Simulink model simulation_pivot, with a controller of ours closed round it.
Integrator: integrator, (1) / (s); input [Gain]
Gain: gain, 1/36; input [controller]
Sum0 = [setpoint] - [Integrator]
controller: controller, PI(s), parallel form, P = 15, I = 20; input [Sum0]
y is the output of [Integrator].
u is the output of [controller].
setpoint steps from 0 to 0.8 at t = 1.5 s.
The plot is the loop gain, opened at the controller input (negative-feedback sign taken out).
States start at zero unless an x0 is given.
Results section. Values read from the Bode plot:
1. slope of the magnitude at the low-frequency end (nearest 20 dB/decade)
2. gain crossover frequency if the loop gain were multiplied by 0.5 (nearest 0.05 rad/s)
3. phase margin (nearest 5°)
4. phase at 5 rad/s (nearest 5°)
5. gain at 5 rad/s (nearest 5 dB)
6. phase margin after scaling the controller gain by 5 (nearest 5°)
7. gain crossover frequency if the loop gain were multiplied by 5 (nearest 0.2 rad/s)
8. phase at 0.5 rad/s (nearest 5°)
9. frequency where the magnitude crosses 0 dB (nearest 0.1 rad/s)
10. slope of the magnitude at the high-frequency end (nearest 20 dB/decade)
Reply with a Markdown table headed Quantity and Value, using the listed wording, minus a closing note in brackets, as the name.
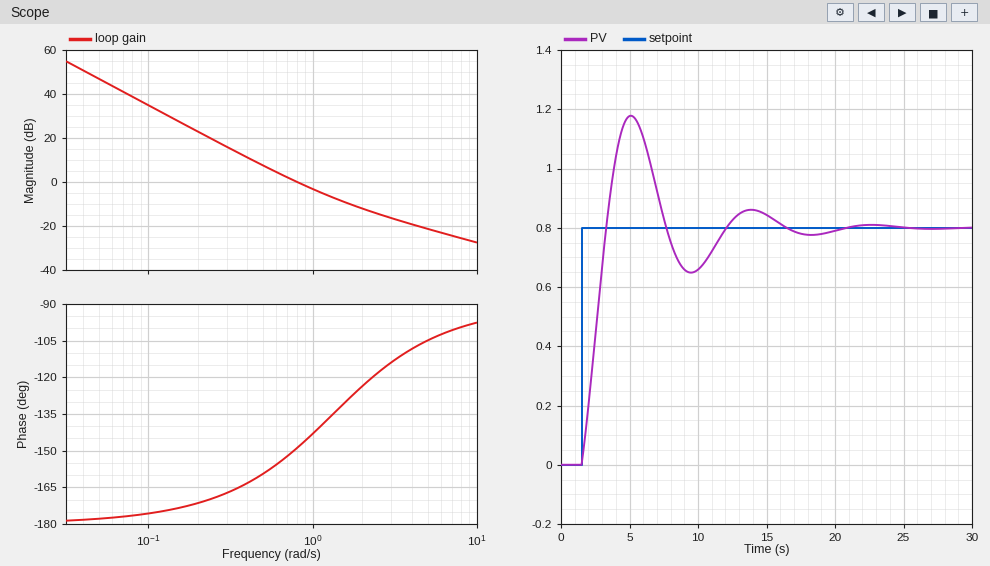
| Quantity | Value |
|---|---|
| slope of the magnitude at the low-frequency end | -40 dB/decade |
| gain crossover frequency if the loop gain were multiplied by 0.5 | 0.55 rad/s |
| phase margin | 30° |
| phase at 5 rad/s | -105° |
| gain at 5 rad/s | -20 dB |
| phase margin after scaling the controller gain by 5 | 60° |
| gain crossover frequency if the loop gain were multiplied by 5 | 2.4 rad/s |
| phase at 0.5 rad/s | -160° |
| frequency where the magnitude crosses 0 dB | 0.8 rad/s |
| slope of the magnitude at the high-frequency end | -20 dB/decade |
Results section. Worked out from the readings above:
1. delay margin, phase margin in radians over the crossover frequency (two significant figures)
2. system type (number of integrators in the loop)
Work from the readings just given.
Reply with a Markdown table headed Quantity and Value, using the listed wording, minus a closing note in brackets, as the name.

| Quantity | Value |
|---|---|
| delay margin, phase margin in radians over the crossover frequency | 0.65 s |
| system type | 2 |
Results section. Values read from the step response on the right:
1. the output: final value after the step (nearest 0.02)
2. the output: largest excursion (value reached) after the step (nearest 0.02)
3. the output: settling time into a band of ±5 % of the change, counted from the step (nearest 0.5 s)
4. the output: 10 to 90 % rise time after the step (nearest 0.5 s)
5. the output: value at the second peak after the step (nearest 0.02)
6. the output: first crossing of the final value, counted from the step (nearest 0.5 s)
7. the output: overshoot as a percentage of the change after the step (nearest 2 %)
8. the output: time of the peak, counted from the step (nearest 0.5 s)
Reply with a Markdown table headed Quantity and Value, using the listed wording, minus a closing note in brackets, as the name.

| Quantity | Value |
|---|---|
| the output: final value after the step | 0.80 |
| the output: largest excursion (value reached) after the step | 1.18 |
| the output: settling time into a band of ±5 % of the change, counted from the step | 13.5 s |
| the output: 10 to 90 % rise time after the step | 1.5 s |
| the output: value at the second peak after the step | 0.86 |
| the output: first crossing of the final value, counted from the step | 2.0 s |
| the output: overshoot as a percentage of the change after the step | 48 % |
| the output: time of the peak, counted from the step | 3.5 s |
